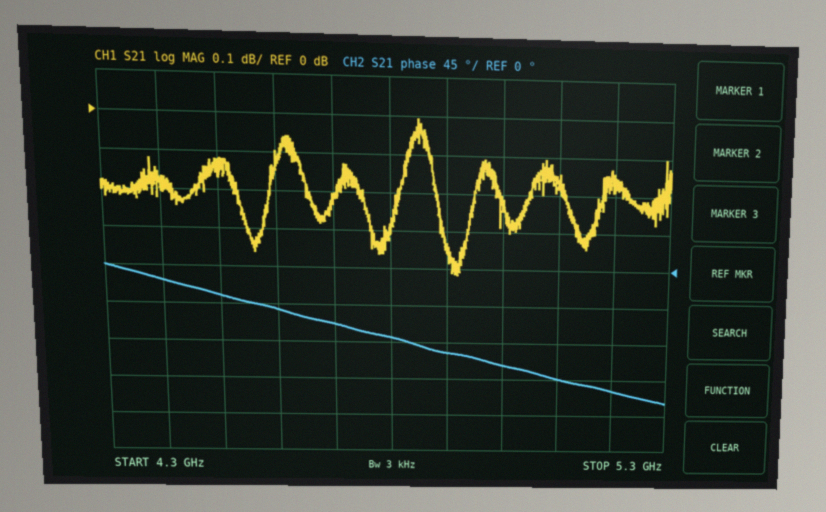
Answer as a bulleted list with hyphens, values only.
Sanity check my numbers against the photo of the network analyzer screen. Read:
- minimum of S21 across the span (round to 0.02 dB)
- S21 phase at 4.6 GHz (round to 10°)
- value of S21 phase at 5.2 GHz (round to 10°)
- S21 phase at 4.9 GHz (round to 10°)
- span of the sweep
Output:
- -0.42 dB
- -50°
- -150°
- -100°
- 1 GHz
